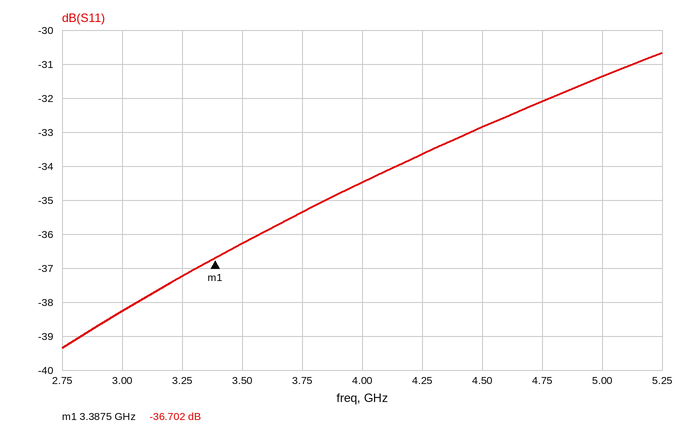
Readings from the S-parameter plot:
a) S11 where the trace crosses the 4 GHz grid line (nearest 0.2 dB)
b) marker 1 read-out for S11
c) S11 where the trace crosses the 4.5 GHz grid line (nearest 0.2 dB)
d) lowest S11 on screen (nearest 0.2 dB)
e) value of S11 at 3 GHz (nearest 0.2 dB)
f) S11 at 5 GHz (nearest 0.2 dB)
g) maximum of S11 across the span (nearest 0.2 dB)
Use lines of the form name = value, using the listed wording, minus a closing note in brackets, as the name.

S11 where the trace crosses the 4 GHz grid line = -34.4 dB
marker 1 read-out for S11 = -36.702 dB
S11 where the trace crosses the 4.5 GHz grid line = -32.8 dB
lowest S11 on screen = -39.4 dB
value of S11 at 3 GHz = -38.2 dB
S11 at 5 GHz = -31.4 dB
maximum of S11 across the span = -30.6 dB
